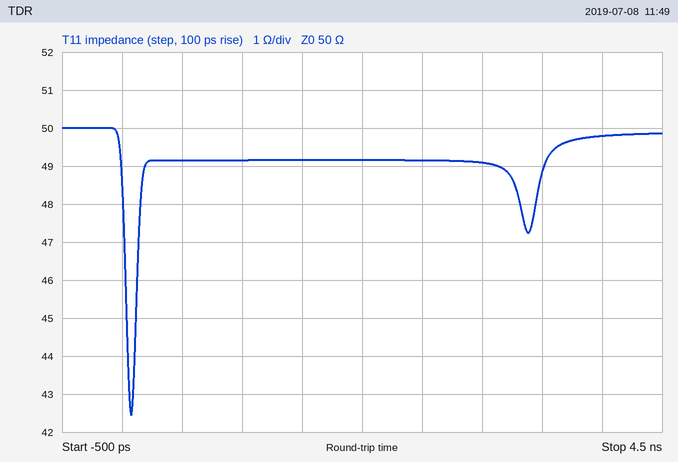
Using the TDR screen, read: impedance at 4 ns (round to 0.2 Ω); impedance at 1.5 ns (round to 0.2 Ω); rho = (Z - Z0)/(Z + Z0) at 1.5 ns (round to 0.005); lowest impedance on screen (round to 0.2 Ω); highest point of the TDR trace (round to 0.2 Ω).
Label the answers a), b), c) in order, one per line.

a) 49.8 Ω
b) 49.2 Ω
c) -0.010
d) 42.4 Ω
e) 50.0 Ω
